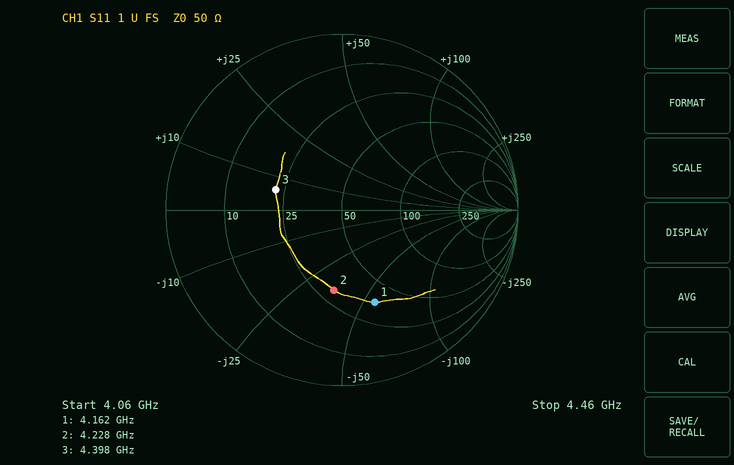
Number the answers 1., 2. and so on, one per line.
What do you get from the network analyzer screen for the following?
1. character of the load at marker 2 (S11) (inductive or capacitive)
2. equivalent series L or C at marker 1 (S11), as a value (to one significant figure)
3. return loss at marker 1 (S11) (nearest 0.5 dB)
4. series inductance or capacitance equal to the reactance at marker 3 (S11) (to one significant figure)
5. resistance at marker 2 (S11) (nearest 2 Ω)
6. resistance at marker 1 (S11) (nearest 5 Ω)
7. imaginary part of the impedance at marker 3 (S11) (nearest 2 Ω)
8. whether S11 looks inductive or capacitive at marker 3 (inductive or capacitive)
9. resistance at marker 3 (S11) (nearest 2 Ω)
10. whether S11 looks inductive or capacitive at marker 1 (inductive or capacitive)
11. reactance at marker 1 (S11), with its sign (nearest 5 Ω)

1. capacitive
2. 700 fF
3. 5.0 dB
4. 200 pH
5. 30 Ω
6. 35 Ω
7. +6 Ω
8. inductive
9. 22 Ω
10. capacitive
11. -55 Ω
